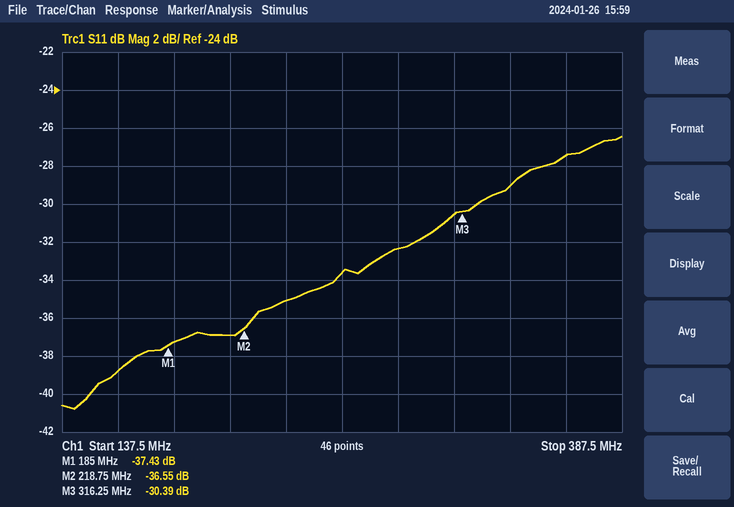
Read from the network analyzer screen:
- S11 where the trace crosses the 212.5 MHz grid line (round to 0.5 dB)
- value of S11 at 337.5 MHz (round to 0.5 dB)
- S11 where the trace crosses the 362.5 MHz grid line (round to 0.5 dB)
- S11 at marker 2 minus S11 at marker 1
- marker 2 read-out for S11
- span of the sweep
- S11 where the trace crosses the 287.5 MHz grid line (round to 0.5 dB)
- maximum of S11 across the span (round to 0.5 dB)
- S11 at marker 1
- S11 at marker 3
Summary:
-37.0 dB
-29.0 dB
-27.5 dB
0.88 dB
-36.55 dB
250 MHz
-32.5 dB
-26.5 dB
-37.43 dB
-30.39 dB
